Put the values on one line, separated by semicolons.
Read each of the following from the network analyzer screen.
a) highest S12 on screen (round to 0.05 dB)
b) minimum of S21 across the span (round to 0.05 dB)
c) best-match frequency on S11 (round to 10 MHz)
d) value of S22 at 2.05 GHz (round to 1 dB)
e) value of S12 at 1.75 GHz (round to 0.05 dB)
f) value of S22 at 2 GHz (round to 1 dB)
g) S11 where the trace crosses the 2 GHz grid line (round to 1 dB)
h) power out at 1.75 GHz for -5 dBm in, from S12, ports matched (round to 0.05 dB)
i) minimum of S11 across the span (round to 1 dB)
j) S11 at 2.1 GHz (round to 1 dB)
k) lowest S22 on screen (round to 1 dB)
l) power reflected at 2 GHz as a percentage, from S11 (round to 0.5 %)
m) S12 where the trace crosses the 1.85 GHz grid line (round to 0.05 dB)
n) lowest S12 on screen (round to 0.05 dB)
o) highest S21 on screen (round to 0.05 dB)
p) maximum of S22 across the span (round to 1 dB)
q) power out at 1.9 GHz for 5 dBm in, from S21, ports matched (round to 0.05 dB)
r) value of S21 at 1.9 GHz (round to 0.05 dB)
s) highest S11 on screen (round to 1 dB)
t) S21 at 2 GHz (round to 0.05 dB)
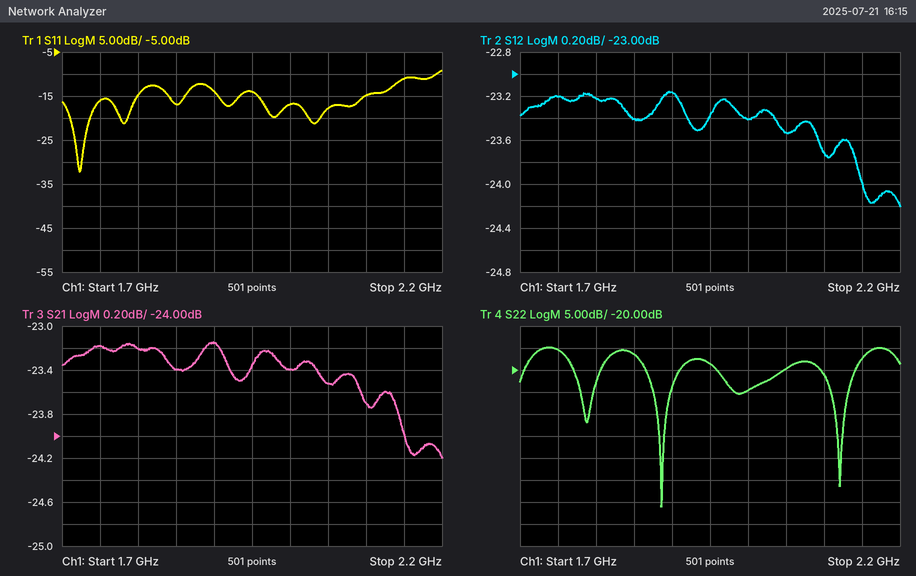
-23.15 dB; -24.20 dB; 1.72 GHz; -20 dB; -23.20 dB; -25 dB; -17 dB; -28.20 dBm; -32 dB; -15 dB; -51 dB; 2.0 %; -23.40 dB; -24.20 dB; -23.15 dB; -15 dB; -18.15 dBm; -23.15 dB; -9 dB; -23.40 dB
